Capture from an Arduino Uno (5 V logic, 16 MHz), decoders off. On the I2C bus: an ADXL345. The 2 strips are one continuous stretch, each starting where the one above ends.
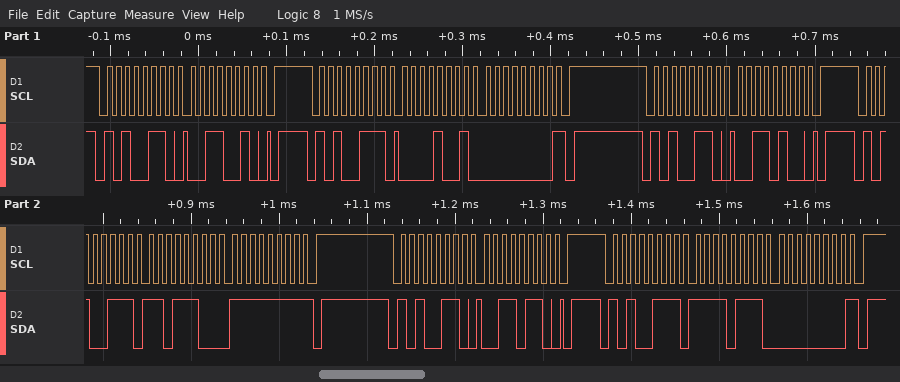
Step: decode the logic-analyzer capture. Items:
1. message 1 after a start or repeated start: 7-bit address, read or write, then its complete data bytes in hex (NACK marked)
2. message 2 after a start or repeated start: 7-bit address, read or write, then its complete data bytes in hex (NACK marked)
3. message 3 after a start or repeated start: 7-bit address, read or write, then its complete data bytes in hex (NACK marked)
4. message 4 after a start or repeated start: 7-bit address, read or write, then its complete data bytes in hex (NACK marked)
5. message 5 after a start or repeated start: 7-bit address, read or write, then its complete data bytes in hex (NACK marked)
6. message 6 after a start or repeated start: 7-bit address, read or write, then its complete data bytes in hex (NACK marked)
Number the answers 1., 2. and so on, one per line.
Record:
1. 0x53 write: 32
2. 0x53 read: 09 00 NACK
3. 0x53 write: 34
4. 0x53 read: DC FF NACK
5. 0x53 write: 36
6. 0x53 read: F7 00 NACK
